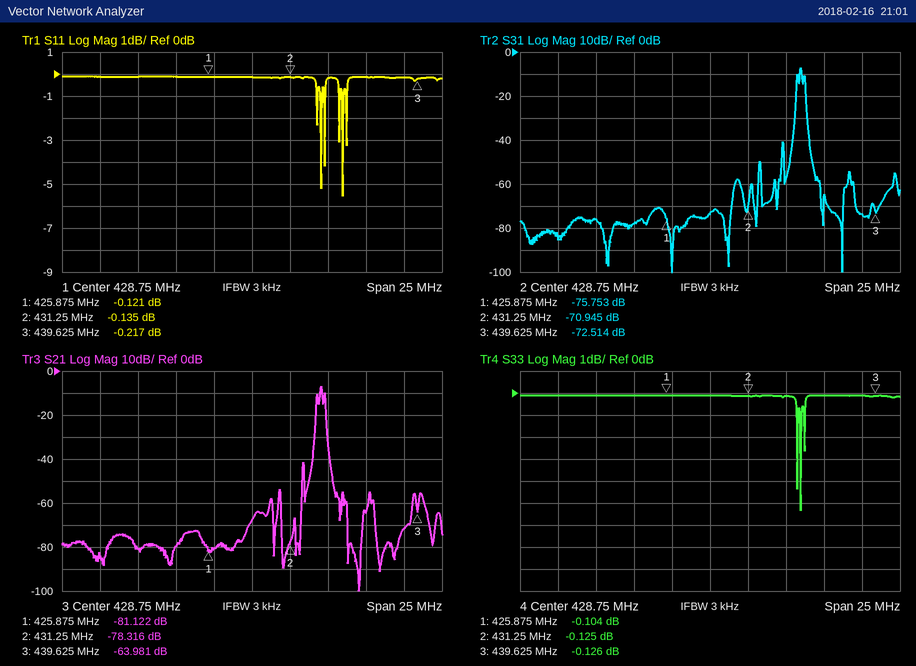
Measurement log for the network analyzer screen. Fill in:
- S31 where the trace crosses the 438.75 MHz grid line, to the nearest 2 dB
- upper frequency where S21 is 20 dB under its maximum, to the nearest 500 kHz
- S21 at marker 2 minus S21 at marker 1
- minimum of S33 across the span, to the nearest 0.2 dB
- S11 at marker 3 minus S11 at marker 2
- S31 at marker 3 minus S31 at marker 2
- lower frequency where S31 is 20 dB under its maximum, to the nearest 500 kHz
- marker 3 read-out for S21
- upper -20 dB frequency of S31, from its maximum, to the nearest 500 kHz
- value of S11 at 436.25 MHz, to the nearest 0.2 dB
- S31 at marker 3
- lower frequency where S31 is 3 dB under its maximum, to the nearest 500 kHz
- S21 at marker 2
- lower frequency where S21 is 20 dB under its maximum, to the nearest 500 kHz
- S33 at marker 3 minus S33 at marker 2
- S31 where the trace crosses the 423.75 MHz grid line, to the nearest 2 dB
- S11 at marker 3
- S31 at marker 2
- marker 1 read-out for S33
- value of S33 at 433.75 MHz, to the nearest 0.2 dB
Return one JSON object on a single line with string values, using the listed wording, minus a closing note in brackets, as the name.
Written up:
{"S31 where the trace crosses the 438.75 MHz grid line, to the nearest 2 dB": "-74 dB", "upper frequency where S21 is 20 dB under its maximum, to the nearest 500 kHz": "433.5 MHz", "S21 at marker 2 minus S21 at marker 1": "2.806 dB", "minimum of S33 across the span, to the nearest 0.2 dB": "-5.4 dB", "S11 at marker 3 minus S11 at marker 2": "-0.082 dB", "S31 at marker 3 minus S31 at marker 2": "-1.569 dB", "lower frequency where S31 is 20 dB under its maximum, to the nearest 500 kHz": "434.5 MHz", "marker 3 read-out for S21": "-63.981 dB", "upper -20 dB frequency of S31, from its maximum, to the nearest 500 kHz": "435.0 MHz", "value of S11 at 436.25 MHz, to the nearest 0.2 dB": "-0.2 dB", "S31 at marker 3": "-72.514 dB", "lower frequency where S31 is 3 dB under its maximum, to the nearest 500 kHz": "434.5 MHz", "S21 at marker 2": "-78.316 dB", "lower frequency where S21 is 20 dB under its maximum, to the nearest 500 kHz": "433.0 MHz", "S33 at marker 3 minus S33 at marker 2": "-0.001 dB", "S31 where the trace crosses the 423.75 MHz grid line, to the nearest 2 dB": "-78 dB", "S11 at marker 3": "-0.217 dB", "S31 at marker 2": "-70.945 dB", "marker 1 read-out for S33": "-0.104 dB", "value of S33 at 433.75 MHz, to the nearest 0.2 dB": "-0.2 dB"}
